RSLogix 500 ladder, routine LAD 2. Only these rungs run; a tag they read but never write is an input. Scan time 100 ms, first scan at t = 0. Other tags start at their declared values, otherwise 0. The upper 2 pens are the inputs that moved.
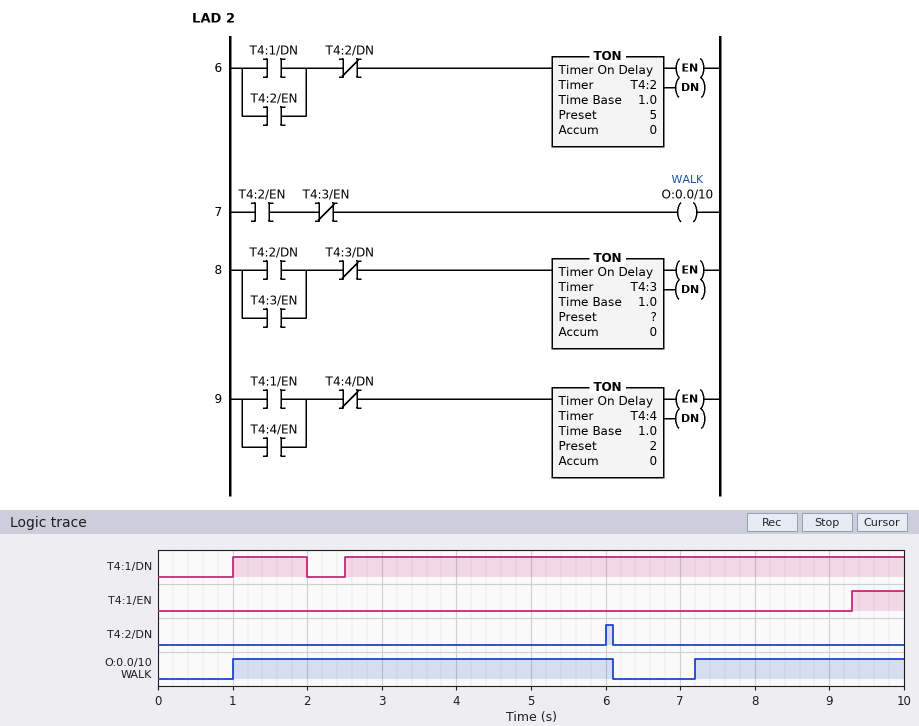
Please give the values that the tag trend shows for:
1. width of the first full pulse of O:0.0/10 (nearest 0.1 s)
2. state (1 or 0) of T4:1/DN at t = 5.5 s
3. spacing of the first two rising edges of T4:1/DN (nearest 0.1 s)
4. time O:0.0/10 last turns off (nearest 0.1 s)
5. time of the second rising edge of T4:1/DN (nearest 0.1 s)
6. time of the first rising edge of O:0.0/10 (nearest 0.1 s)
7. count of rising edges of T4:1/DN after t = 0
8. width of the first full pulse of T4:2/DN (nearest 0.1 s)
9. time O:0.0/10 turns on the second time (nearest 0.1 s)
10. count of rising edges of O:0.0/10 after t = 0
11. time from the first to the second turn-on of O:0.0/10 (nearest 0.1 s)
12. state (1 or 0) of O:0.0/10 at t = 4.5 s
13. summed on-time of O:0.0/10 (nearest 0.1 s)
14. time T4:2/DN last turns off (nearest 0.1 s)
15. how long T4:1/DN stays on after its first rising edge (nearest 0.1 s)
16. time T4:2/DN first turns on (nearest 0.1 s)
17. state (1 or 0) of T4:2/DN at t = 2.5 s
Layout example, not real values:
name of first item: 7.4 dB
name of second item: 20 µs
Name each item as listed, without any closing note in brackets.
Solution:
width of the first full pulse of O:0.0/10: 5.1 s
state (1 or 0) of T4:1/DN at t = 5.5 s: 1
spacing of the first two rising edges of T4:1/DN: 1.5 s
time O:0.0/10 last turns off: 6.1 s
time of the second rising edge of T4:1/DN: 2.5 s
time of the first rising edge of O:0.0/10: 1.0 s
count of rising edges of T4:1/DN after t = 0: 2
width of the first full pulse of T4:2/DN: 0.1 s
time O:0.0/10 turns on the second time: 7.2 s
count of rising edges of O:0.0/10 after t = 0: 2
time from the first to the second turn-on of O:0.0/10: 6.2 s
state (1 or 0) of O:0.0/10 at t = 4.5 s: 1
summed on-time of O:0.0/10: 7.9 s
time T4:2/DN last turns off: 6.1 s
how long T4:1/DN stays on after its first rising edge: 1.0 s
time T4:2/DN first turns on: 6.0 s
state (1 or 0) of T4:2/DN at t = 2.5 s: 0
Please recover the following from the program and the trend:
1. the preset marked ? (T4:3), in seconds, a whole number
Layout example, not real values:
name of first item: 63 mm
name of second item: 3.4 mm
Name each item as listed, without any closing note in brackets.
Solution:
the preset marked ? (T4:3), in seconds, a whole number: 1 s
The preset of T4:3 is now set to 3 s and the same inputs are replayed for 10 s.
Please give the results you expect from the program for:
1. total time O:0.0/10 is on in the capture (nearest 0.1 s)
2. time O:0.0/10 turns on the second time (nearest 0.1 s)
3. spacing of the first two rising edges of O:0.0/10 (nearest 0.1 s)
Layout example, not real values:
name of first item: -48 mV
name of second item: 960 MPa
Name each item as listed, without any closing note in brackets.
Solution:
total time O:0.0/10 is on in the capture: 5.9 s
time O:0.0/10 turns on the second time: 9.2 s
spacing of the first two rising edges of O:0.0/10: 8.2 s
